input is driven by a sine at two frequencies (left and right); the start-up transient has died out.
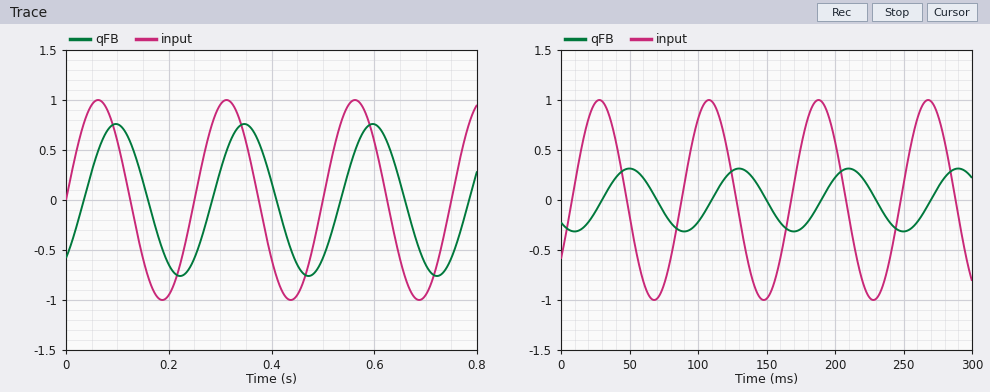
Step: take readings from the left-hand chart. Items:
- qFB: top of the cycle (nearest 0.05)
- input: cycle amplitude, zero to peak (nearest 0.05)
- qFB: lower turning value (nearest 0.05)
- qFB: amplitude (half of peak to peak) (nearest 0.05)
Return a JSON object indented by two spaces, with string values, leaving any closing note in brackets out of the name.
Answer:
{
  "qFB: top of the cycle": "0.75",
  "input: cycle amplitude, zero to peak": "1.00",
  "qFB: lower turning value": "-0.75",
  "qFB: amplitude (half of peak to peak)": "0.75"
}
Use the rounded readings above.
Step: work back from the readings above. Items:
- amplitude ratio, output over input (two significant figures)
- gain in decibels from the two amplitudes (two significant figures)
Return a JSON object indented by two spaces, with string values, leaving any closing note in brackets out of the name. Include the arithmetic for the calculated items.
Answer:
{
  "amplitude ratio, output over input": "0.75 / 1 = 0.75",
  "gain in decibels from the two amplitudes": "20 log10(0.75 / 1) = -2.5 dB"
}
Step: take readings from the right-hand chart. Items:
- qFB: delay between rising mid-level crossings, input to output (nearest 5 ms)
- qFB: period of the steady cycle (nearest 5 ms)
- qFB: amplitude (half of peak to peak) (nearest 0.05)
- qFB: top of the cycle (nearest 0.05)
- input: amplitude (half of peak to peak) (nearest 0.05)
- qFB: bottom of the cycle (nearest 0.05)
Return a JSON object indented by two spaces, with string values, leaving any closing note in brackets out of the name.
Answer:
{
  "qFB: delay between rising mid-level crossings, input to output": "20 ms",
  "qFB: period of the steady cycle": "80 ms",
  "qFB: amplitude (half of peak to peak)": "0.30",
  "qFB: top of the cycle": "0.30",
  "input: amplitude (half of peak to peak)": "1.00",
  "qFB: bottom of the cycle": "-0.30"
}
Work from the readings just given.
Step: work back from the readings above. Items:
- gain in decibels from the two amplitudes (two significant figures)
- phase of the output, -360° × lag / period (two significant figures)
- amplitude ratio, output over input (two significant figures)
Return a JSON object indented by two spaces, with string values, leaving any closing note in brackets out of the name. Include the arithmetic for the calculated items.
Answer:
{
  "gain in decibels from the two amplitudes": "20 log10(0.3 / 1) = -10 dB",
  "phase of the output, -360° × lag / period": "-360 × 20 / 80 = -90°",
  "amplitude ratio, output over input": "0.3 / 1 = 0.30"
}
